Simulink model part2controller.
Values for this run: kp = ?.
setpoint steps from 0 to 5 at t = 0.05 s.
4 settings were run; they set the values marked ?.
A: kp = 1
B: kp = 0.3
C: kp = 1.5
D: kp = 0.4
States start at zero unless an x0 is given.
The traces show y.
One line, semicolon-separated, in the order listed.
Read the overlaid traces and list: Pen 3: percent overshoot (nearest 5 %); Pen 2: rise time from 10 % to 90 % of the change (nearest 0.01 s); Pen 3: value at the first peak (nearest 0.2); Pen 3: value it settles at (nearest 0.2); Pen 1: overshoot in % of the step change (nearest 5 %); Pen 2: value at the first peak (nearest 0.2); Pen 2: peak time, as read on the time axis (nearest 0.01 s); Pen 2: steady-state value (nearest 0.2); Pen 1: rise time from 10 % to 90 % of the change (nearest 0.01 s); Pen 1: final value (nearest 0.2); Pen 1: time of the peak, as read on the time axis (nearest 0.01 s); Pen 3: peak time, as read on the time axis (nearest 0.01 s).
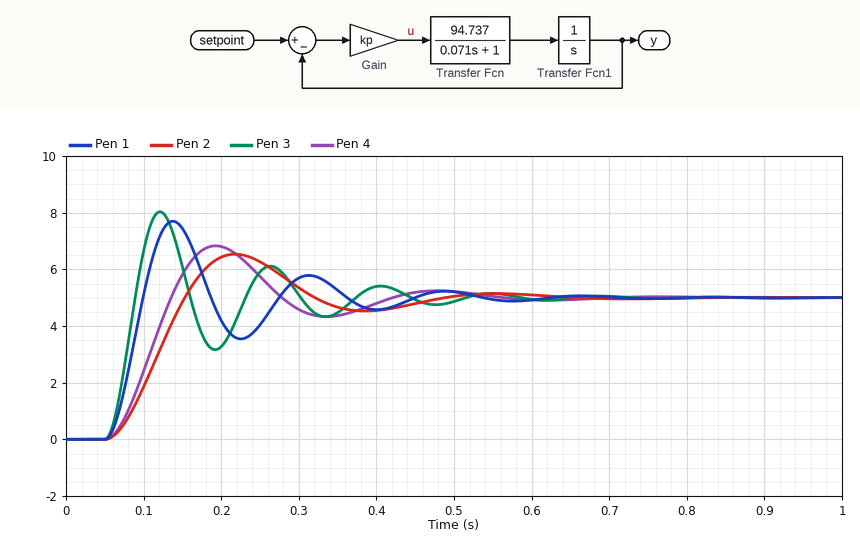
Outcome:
60 %; 0.07 s; 8.0; 5.0; 55 %; 6.6; 0.22 s; 5.0; 0.03 s; 5.0; 0.14 s; 0.12 s
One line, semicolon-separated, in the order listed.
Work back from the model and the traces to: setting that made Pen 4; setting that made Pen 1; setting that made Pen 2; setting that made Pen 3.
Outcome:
D; A; B; C
